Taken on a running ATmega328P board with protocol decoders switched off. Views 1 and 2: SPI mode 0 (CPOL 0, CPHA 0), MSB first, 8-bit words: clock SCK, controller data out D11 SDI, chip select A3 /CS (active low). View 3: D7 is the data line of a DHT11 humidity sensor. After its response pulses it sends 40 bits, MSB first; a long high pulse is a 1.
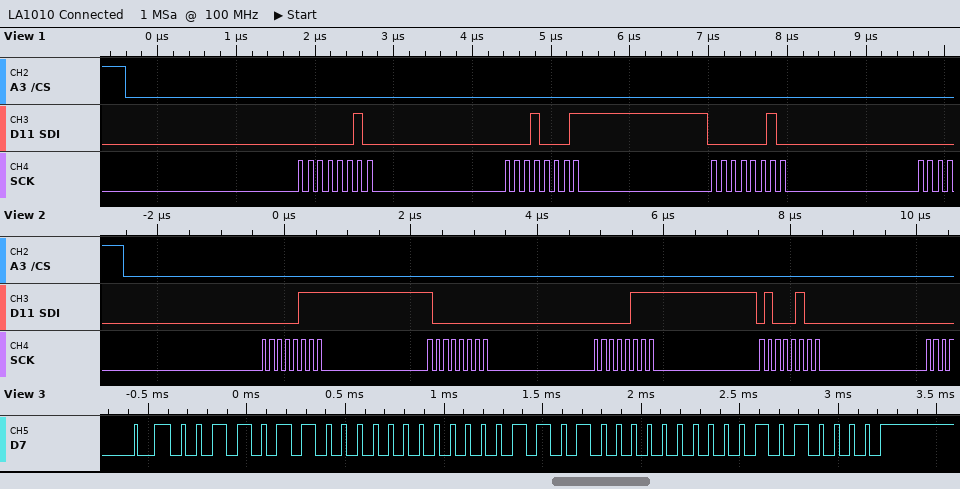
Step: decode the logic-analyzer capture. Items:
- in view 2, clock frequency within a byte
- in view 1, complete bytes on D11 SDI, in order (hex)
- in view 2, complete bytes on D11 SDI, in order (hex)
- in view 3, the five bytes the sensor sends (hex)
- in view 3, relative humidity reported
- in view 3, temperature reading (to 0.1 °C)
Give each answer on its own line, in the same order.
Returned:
8 MHz
0x02 0x11 0x02
07 80 07 44
36 00 1A 00 50
54 %
26.0 °C
